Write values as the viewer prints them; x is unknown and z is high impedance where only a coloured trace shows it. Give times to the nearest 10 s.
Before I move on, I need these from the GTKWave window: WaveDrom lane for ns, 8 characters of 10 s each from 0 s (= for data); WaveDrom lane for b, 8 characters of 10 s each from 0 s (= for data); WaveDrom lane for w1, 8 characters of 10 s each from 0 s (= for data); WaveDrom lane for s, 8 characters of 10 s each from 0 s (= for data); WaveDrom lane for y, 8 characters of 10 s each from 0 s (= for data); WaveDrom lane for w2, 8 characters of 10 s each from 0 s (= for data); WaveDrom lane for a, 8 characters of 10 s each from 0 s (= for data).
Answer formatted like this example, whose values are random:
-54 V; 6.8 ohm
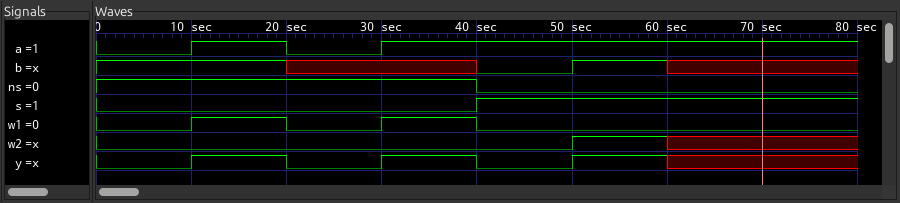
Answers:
{name: 'ns', wave: '1...0...'}; {name: 'b', wave: '1.x.01x.'}; {name: 'w1', wave: '01010...'}; {name: 's', wave: '0...1...'}; {name: 'y', wave: '010101x.'}; {name: 'w2', wave: '0....1x.'}; {name: 'a', wave: '0101....'}
